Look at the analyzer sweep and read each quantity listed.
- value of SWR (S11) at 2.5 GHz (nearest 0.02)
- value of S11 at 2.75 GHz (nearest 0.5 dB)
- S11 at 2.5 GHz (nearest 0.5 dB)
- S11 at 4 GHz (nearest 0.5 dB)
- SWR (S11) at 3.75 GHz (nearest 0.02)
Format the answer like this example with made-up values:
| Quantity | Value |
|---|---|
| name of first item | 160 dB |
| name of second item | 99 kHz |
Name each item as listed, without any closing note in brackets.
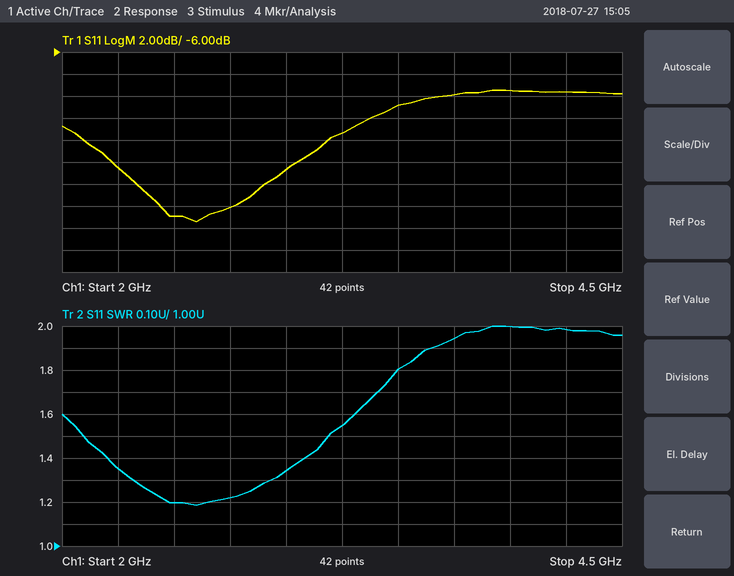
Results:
| Quantity | Value |
|---|---|
| value of SWR (S11) at 2.5 GHz | 1.20 |
| value of S11 at 2.75 GHz | -20.0 dB |
| S11 at 2.5 GHz | -21.0 dB |
| S11 at 4 GHz | -9.5 dB |
| SWR (S11) at 3.75 GHz | 1.94 |
